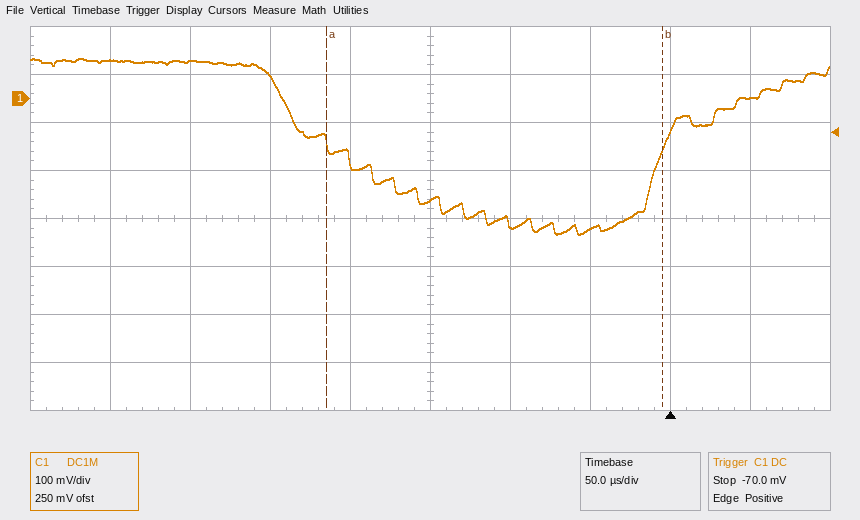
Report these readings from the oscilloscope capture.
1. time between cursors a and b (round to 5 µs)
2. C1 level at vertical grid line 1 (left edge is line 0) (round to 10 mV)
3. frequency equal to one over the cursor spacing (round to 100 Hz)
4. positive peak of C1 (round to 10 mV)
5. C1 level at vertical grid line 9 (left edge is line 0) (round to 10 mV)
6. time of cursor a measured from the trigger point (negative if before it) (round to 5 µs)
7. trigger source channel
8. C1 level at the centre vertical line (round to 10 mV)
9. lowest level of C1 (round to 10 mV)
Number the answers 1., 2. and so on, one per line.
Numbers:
1. 210 µs
2. 80 mV
3. 4.8 kHz
4. 80 mV
5. 0 mV
6. -215 µs
7. C1
8. -210 mV
9. -280 mV
